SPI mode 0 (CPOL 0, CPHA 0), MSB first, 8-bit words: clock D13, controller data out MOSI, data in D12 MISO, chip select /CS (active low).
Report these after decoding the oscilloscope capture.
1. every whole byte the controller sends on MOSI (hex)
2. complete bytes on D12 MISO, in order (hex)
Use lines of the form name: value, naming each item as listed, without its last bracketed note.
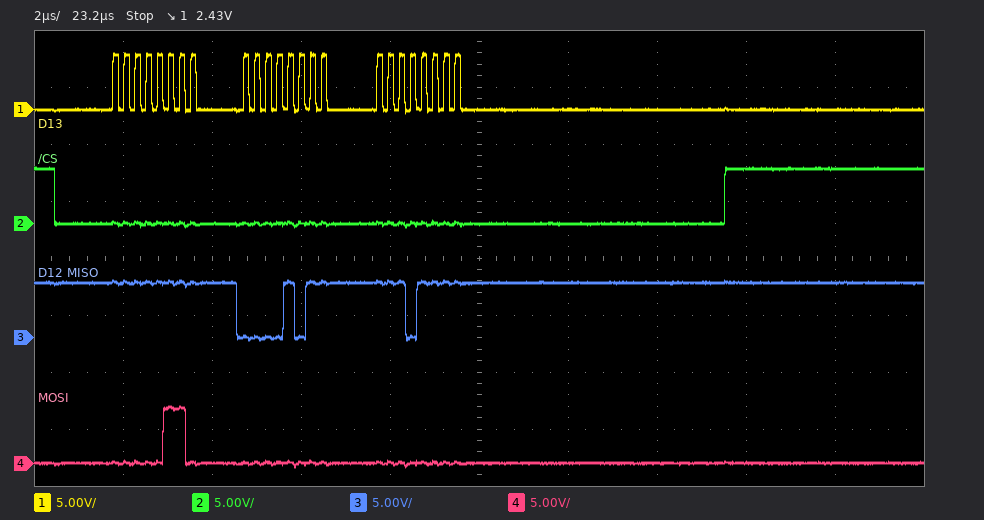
every whole byte the controller sends on MOSI: 06 00 00
complete bytes on D12 MISO, in order: FF 0B EF
